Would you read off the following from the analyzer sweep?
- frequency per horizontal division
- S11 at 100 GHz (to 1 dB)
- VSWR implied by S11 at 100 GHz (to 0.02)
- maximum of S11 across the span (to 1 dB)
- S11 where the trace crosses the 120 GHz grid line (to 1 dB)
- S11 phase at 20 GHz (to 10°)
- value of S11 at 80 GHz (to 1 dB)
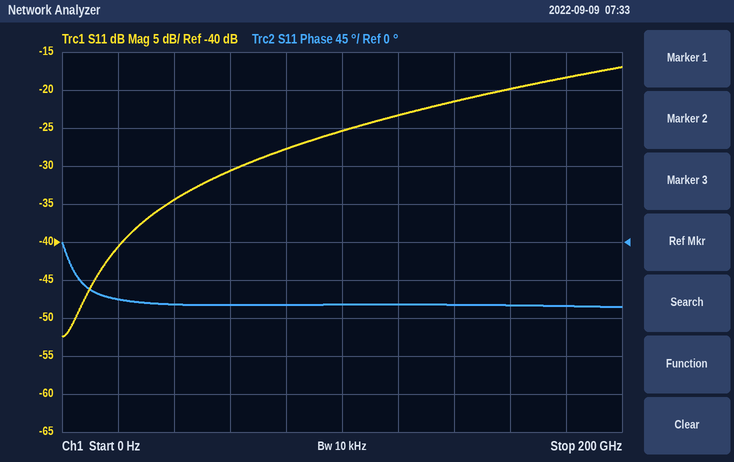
20 GHz
-25 dB
1.12
-17 dB
-23 dB
-70°
-28 dB
